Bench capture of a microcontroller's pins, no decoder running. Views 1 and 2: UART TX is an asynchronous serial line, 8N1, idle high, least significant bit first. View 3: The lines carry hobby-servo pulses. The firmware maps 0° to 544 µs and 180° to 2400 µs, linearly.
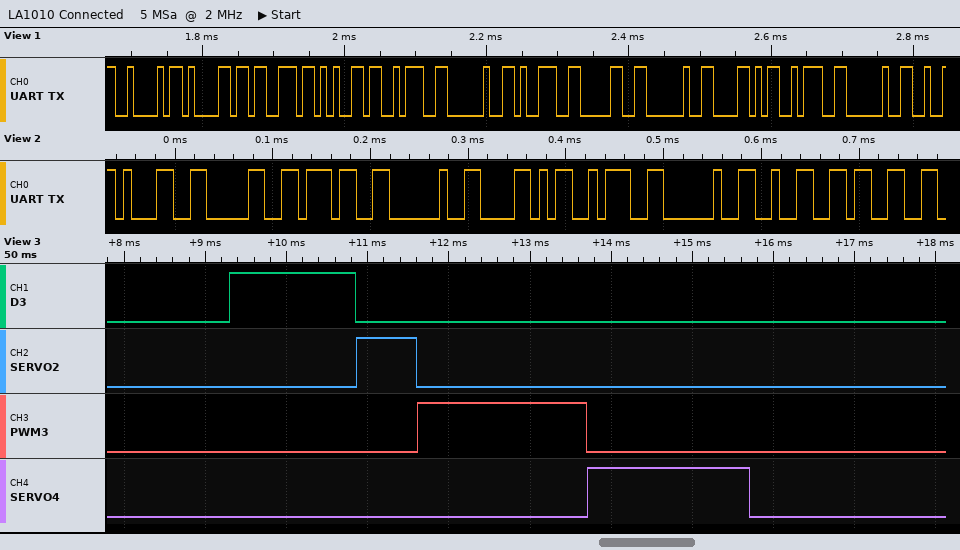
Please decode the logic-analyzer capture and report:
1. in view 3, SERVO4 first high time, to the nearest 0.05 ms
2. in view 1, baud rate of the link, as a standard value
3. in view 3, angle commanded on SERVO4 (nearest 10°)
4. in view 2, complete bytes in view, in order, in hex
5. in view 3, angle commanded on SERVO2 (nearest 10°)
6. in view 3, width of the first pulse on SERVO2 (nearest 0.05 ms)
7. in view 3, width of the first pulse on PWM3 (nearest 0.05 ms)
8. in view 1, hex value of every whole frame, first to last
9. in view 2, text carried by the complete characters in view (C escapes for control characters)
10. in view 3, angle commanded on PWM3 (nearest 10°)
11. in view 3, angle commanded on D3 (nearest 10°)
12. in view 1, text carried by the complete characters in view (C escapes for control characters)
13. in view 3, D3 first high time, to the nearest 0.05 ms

2.00 ms
115200 baud
140°
31 30 37 20 58 3A 20 32 33
20°
0.75 ms
2.10 ms
0x42 0x61 0x73 0x65 0x3A 0x20 0x39 0x30 0x20 0x58 0x3A 0x20
"107 X: 23"
150°
100°
"Base: 90 X: "
1.55 ms
